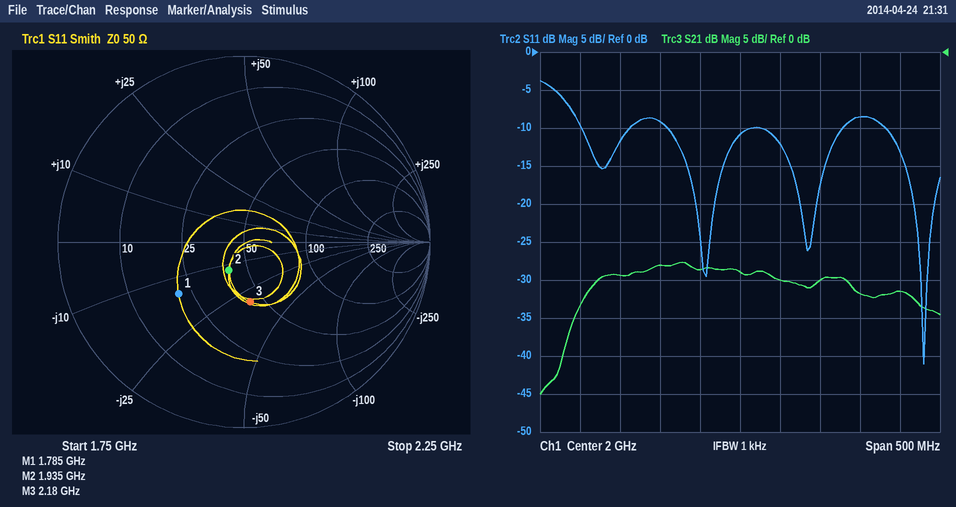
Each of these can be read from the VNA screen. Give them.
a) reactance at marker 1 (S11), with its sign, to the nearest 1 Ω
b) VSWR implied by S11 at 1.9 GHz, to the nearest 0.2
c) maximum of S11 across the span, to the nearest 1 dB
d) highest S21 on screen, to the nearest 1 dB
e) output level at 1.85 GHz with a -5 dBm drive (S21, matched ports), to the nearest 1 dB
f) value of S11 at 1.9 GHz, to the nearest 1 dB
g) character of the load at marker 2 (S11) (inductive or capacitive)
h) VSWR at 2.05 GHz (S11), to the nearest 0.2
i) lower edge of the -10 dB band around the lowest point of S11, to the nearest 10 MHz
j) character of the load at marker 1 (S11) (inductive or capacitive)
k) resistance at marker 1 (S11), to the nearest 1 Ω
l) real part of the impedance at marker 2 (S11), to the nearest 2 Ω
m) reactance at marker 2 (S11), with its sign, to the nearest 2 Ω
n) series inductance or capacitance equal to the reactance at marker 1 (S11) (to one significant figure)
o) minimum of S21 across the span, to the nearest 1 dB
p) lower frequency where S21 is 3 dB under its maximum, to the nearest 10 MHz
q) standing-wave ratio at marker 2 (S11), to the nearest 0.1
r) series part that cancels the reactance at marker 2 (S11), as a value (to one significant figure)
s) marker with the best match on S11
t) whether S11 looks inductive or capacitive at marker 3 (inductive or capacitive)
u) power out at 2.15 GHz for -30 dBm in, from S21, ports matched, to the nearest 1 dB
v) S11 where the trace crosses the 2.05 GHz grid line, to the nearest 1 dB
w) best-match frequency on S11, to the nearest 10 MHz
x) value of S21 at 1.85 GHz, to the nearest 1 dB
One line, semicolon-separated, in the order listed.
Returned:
-15 Ω; 2.0; -4 dB; -28 dB; -34 dBm; -9 dB; capacitive; 1.6; 2.18 GHz; capacitive; 21 Ω; 40 Ω; -12 Ω; 6 pF; -45 dB; 1.82 GHz; 1.4; 1 nH; marker 2; capacitive; -62 dBm; -12 dB; 2.23 GHz; -29 dB
